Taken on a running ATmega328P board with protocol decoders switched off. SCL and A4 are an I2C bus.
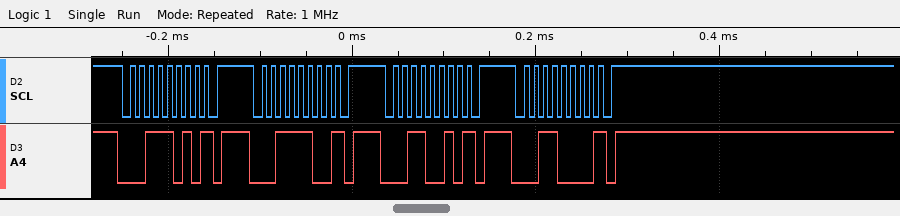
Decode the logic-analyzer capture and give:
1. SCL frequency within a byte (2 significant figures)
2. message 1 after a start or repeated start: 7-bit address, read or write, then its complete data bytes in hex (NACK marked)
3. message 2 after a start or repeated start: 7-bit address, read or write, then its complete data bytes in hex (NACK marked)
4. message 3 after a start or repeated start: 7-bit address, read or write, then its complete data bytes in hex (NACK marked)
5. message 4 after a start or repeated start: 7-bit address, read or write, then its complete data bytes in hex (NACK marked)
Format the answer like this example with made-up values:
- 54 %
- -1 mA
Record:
- 100 kHz
- 0x1D write NACK
- 0x1E write NACK
- 0x19 write NACK
- 0x18 write NACK
